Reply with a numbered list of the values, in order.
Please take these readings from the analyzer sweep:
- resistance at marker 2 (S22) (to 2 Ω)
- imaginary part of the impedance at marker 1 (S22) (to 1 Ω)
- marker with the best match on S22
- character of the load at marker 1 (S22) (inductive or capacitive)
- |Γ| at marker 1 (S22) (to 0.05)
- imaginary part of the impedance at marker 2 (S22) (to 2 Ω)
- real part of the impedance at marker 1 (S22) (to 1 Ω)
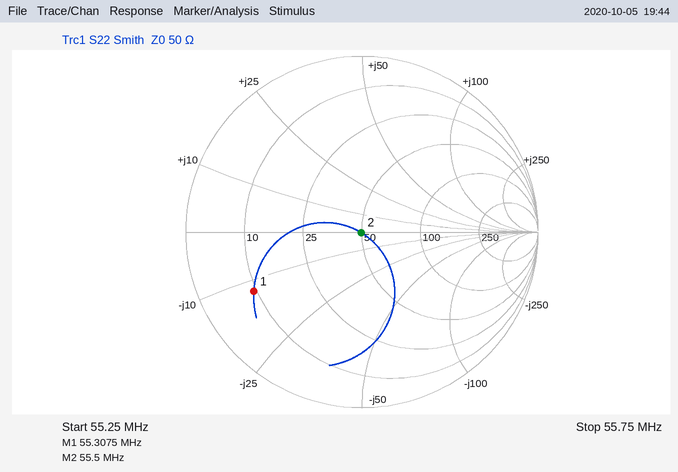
1. 50 Ω
2. -12 Ω
3. marker 2
4. capacitive
5. 0.70
6. 0 Ω
7. 9 Ω
